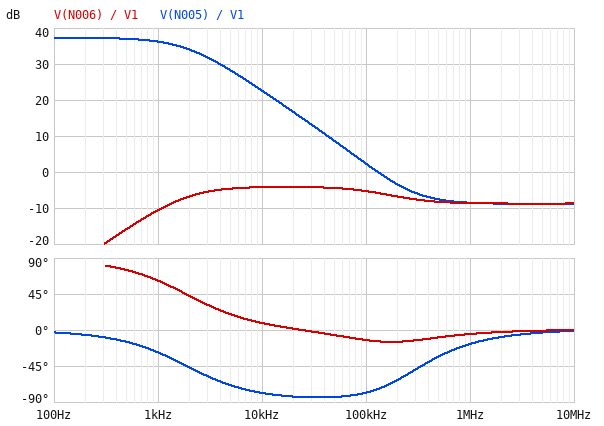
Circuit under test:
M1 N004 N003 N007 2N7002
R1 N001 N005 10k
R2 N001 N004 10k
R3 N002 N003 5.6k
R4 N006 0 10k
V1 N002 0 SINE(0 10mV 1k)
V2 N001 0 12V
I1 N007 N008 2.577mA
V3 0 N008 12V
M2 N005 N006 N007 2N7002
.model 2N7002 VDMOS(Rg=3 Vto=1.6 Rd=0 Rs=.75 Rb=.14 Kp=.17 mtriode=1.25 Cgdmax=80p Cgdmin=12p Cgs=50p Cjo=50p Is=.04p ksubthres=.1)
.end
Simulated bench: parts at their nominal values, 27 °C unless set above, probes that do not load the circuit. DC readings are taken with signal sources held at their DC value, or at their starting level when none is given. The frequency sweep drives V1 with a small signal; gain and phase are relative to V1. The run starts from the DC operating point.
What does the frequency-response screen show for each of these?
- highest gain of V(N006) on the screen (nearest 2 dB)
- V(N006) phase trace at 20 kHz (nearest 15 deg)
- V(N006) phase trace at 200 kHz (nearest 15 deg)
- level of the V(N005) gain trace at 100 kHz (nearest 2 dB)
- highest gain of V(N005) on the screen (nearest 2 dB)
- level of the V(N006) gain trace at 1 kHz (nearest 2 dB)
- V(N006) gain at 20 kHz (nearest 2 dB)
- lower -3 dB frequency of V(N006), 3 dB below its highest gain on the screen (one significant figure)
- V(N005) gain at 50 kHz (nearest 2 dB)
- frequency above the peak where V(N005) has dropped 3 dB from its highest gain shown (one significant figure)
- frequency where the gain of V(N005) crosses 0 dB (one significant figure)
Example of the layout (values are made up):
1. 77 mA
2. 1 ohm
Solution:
1. -4 dB
2. 0 deg
3. -15 deg
4. 2 dB
5. 38 dB
6. -10 dB
7. -4 dB
8. 2 kHz
9. 8 dB
10. 2 kHz
11. 100 kHz
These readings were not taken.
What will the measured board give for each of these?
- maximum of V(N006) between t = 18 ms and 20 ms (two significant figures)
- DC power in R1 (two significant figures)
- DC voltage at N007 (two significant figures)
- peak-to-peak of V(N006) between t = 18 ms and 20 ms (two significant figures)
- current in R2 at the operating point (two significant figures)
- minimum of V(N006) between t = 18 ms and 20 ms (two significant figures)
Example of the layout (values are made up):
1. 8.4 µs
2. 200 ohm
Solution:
1. 3.0 mV
2. 17 mW
3. -1.7 V
4. 5.9 mV
5. 1.3 mA
6. -2.9 mV
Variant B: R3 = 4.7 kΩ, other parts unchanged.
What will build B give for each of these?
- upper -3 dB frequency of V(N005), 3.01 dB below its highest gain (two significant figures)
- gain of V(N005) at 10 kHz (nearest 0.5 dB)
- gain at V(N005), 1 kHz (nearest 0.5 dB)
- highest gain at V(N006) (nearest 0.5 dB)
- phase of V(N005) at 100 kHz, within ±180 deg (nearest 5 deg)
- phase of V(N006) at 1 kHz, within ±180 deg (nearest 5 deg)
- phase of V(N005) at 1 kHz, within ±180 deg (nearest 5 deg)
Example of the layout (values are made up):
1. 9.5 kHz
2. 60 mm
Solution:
1. 2.0 kHz
2. 23.0 dB
3. 36.5 dB
4. -3.5 dB
5. -75 deg
6. 65 deg
7. -25 deg
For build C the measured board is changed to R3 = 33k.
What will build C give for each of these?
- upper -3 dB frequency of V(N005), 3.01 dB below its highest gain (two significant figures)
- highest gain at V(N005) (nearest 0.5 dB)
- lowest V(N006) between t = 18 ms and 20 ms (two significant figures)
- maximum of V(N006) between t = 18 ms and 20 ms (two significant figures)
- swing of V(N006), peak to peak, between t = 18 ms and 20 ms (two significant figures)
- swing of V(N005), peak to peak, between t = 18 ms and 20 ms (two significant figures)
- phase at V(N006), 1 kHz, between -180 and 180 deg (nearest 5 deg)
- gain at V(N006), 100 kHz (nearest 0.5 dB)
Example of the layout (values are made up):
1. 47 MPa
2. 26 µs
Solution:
1. 690 Hz
2. 37.5 dB
3. -1.9 mV
4. 1.9 mV
5. 3.8 mV
6. 830 mV
7. 35 deg
8. -15.5 dB
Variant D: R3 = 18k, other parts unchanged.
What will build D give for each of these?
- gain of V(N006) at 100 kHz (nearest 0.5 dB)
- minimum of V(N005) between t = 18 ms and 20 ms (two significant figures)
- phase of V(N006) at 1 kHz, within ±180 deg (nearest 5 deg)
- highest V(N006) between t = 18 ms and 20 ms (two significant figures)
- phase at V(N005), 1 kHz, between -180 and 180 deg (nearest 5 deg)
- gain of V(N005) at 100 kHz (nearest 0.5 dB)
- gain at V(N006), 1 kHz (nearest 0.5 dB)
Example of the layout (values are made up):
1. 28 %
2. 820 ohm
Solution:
1. -11.5 dB
2. -1.4 V
3. 45 deg
4. 2.4 mV
5. -45 deg
6. -4.0 dB
7. -12.5 dB
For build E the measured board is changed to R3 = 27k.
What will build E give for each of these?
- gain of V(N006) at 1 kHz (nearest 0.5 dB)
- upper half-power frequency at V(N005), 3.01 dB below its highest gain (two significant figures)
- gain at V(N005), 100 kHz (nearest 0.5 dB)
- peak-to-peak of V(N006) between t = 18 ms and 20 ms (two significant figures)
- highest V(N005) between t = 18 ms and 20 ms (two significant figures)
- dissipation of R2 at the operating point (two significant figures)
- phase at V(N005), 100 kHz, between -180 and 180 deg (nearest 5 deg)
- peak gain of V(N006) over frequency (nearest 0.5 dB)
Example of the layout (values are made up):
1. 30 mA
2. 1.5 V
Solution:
1. -13.5 dB
2. 800 Hz
3. -6.5 dB
4. 4.2 mV
5. -430 mV
6. 17 mW
7. -90 deg
8. -11.5 dB
